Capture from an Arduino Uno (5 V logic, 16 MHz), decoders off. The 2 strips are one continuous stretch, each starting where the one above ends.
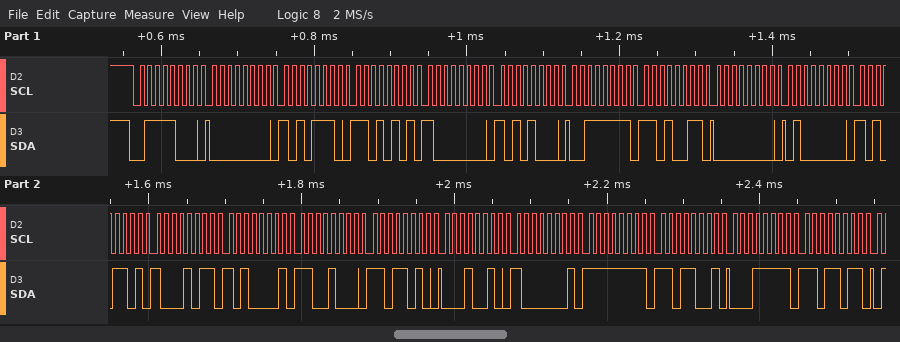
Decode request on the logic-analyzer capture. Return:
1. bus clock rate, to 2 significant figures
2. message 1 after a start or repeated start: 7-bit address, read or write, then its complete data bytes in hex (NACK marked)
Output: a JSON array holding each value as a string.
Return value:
["100 kHz", "0x3C write: 00 AE D5 80 A8 3F D3 00 40 AD 8B A1 C8 DA 12 81 FF D9 1F DB"]
